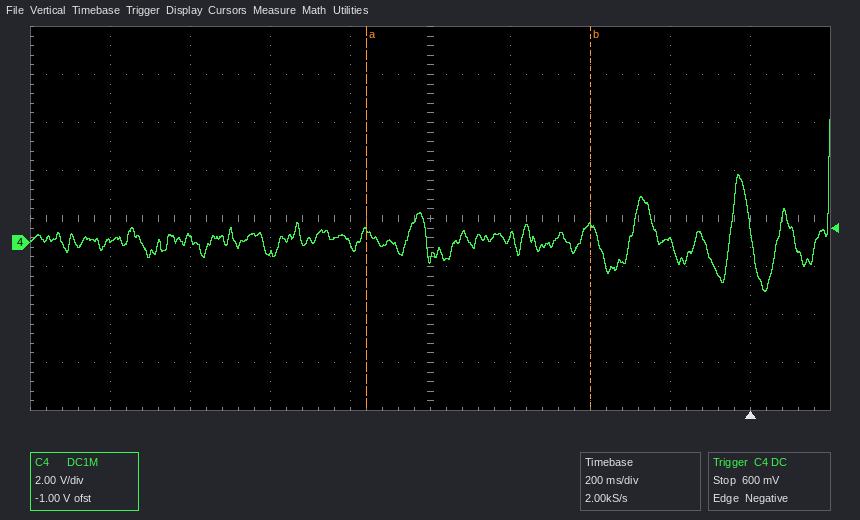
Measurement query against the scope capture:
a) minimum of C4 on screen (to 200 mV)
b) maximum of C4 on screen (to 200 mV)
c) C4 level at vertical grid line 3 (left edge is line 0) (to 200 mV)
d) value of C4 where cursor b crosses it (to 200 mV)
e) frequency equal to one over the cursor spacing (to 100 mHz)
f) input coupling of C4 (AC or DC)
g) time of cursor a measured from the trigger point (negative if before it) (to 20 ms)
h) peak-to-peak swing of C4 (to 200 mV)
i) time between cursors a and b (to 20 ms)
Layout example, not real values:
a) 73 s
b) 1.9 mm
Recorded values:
a) -2.0 V
b) 5.2 V
c) -400 mV
d) 800 mV
e) 1.8 Hz
f) DC
g) -960 ms
h) 7.2 V
i) 560 ms
